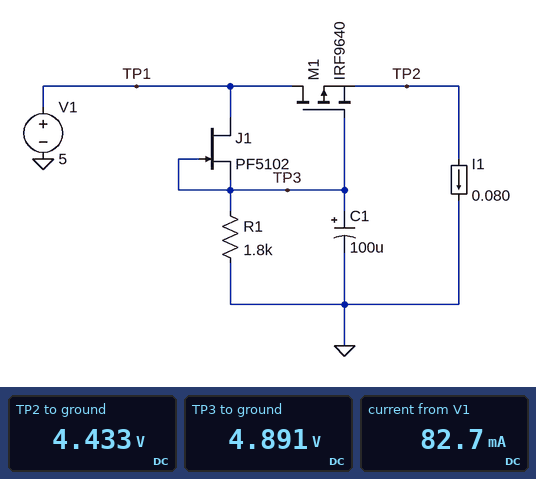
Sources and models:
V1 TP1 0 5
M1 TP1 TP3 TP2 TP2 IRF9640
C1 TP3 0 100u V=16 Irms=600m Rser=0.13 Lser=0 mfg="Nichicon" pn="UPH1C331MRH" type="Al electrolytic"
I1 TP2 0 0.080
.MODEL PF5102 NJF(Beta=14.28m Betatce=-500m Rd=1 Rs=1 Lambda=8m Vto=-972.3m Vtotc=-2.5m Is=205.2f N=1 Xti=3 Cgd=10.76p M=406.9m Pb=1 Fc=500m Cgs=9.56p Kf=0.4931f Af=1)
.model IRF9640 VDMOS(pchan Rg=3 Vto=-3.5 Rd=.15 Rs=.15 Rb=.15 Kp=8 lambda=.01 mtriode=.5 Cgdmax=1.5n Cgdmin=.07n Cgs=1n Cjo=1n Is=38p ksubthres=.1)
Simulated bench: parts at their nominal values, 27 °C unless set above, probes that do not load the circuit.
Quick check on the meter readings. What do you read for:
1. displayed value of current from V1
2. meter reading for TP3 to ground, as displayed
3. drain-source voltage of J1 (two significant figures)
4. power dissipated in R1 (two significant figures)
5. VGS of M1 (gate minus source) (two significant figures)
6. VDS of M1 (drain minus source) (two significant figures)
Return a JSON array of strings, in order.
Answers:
["82.7 mA", "4.891 V", "110 mV", "13 mW", "460 mV", "570 mV"]
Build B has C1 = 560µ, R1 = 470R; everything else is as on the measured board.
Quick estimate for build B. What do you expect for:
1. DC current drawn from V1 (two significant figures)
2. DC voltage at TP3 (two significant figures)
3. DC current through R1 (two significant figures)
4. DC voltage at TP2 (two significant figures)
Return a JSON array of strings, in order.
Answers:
["90 mA", "4.5 V", "9.6 mA", "4.4 V"]
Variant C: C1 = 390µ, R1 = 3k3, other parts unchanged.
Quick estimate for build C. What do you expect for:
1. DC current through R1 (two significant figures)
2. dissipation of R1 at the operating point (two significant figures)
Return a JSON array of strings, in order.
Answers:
["1.5 mA", "7.4 mW"]
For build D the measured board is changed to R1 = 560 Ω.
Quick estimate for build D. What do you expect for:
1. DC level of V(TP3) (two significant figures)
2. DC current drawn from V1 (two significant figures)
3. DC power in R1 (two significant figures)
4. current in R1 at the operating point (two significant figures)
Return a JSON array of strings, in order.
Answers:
["4.6 V", "88 mA", "38 mW", "8.2 mA"]
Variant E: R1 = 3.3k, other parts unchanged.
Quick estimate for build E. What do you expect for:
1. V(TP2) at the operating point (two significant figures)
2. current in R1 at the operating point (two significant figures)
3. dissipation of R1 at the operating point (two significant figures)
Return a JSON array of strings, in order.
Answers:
["4.4 V", "1.5 mA", "7.4 mW"]
